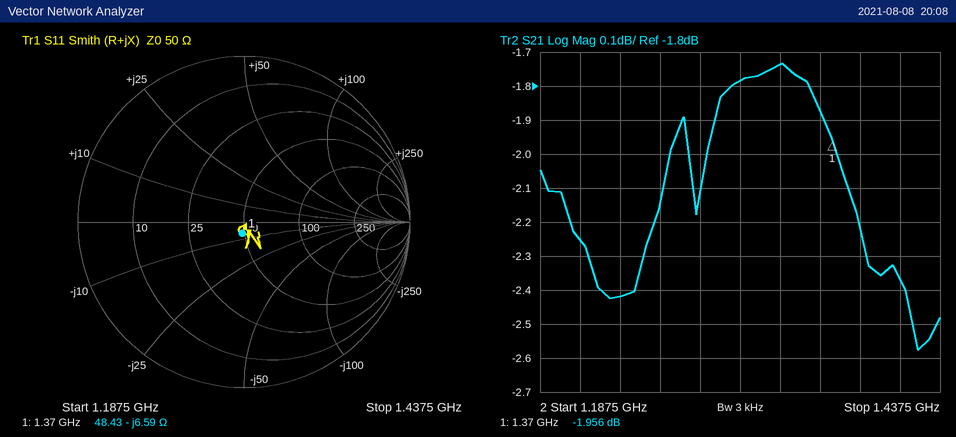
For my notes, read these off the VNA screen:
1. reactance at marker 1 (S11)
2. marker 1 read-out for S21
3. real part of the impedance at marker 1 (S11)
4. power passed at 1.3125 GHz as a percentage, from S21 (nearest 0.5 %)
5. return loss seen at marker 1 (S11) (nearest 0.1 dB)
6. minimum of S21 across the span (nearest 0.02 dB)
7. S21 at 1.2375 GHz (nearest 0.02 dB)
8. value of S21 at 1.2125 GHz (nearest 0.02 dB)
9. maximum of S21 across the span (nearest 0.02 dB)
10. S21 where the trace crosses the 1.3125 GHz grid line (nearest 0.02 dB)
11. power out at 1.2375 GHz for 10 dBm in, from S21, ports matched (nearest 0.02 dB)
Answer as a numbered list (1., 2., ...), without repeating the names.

1. -6.59 Ω
2. -1.956 dB
3. 48.43 Ω
4. 66.5 %
5. 23.3 dB
6. -2.58 dB
7. -2.42 dB
8. -2.26 dB
9. -1.74 dB
10. -1.78 dB
11. 7.58 dBm
